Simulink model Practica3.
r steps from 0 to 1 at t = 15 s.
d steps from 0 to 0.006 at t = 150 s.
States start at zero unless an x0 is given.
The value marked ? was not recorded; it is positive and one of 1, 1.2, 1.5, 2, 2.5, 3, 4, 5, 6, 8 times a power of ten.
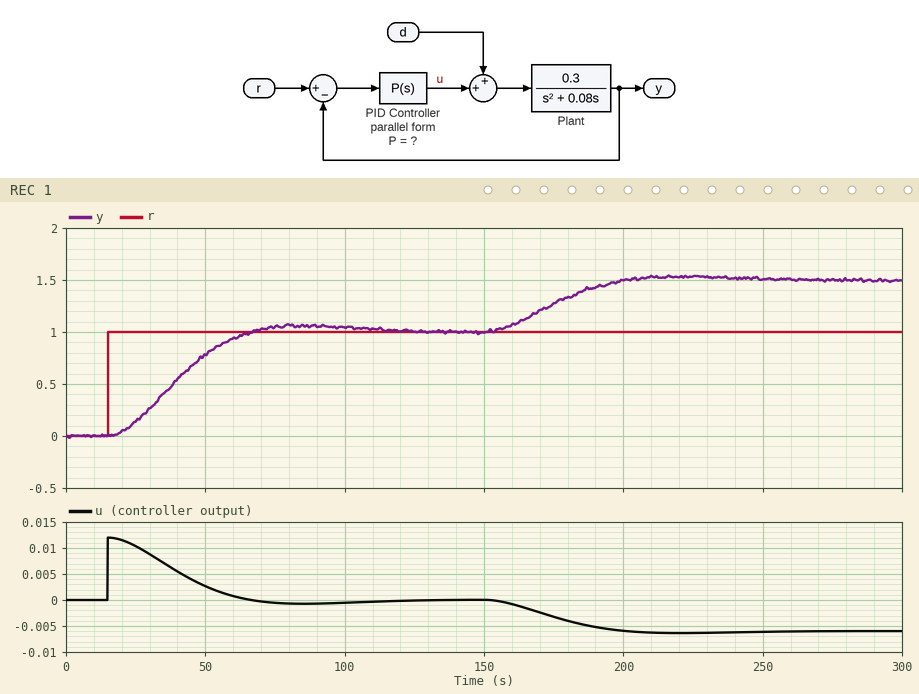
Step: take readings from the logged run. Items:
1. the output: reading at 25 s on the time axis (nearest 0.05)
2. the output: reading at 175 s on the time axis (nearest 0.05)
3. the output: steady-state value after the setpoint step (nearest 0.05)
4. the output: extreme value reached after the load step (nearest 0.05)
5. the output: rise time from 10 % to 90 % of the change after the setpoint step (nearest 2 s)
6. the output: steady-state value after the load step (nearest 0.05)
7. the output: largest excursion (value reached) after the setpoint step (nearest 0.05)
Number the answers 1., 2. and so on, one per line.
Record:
1. 0.15
2. 1.25
3. 1.00
4. 1.55
5. 34 s
6. 1.50
7. 1.05
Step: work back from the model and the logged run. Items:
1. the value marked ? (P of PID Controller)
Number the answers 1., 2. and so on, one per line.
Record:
1. 0.012
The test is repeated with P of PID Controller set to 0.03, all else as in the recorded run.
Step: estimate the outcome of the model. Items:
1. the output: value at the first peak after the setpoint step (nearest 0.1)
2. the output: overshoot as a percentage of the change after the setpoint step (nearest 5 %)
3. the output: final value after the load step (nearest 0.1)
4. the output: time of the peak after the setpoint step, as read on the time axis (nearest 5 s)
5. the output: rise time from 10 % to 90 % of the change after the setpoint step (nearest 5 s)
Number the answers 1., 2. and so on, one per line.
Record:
1. 1.2
2. 25 %
3. 1.2
4. 50 s
5. 15 s
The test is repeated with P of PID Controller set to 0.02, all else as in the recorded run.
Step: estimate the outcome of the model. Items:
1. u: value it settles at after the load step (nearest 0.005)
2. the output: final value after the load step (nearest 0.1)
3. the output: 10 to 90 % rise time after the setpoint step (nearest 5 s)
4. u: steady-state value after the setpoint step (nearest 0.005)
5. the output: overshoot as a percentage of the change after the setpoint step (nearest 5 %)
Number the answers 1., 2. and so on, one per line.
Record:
1. -0.005
2. 1.3
3. 20 s
4. 0.000
5. 15 %
